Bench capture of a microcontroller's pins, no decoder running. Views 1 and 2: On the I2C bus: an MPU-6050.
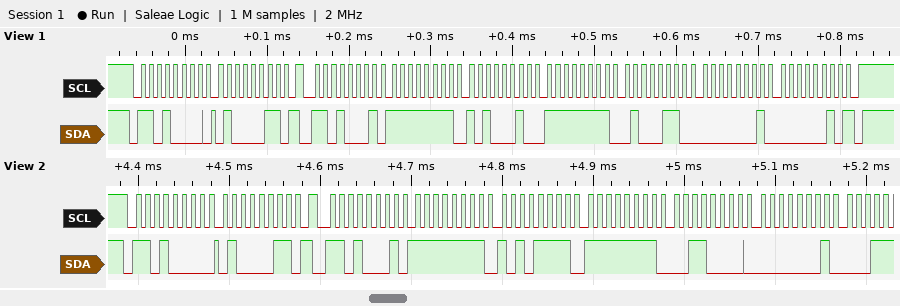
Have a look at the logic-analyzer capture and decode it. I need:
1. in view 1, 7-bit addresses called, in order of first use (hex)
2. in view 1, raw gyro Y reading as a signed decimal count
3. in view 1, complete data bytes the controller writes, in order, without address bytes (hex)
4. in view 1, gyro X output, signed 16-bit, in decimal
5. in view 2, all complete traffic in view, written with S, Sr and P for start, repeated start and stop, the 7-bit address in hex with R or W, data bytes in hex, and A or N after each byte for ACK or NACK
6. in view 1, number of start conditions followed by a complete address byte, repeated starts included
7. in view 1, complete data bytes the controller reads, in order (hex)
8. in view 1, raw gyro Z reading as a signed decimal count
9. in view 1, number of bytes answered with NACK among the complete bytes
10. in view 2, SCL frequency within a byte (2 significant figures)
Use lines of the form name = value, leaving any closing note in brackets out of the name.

in view 1, 7-bit addresses called, in order of first use = 0x68
in view 1, raw gyro Y reading as a signed decimal count = -186
in view 1, complete data bytes the controller writes, in order, without address bytes = 43
in view 1, gyro X output, signed 16-bit, in decimal = -94
in view 2, all complete traffic in view, written with S, Sr and P for start, repeated start and stop, the 7-bit address in hex with R or W, data bytes in hex, and A or N after each byte for ACK or NACK = S 68W A 43 A Sr 68R A FF A AF A FF A 30 A 01 A
in view 1, number of start conditions followed by a complete address byte, repeated starts included = 2
in view 1, complete data bytes the controller reads, in order = FF A2 FF 46 01 02
in view 1, raw gyro Z reading as a signed decimal count = 258
in view 1, number of bytes answered with NACK among the complete bytes = 1
in view 2, SCL frequency within a byte = 100 kHz
